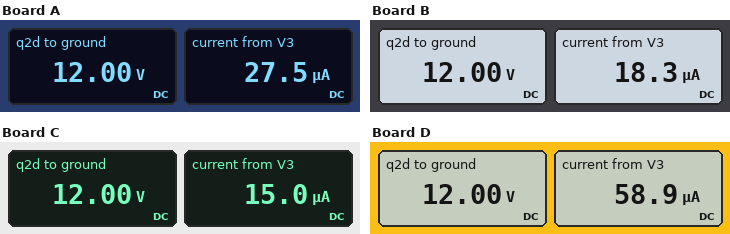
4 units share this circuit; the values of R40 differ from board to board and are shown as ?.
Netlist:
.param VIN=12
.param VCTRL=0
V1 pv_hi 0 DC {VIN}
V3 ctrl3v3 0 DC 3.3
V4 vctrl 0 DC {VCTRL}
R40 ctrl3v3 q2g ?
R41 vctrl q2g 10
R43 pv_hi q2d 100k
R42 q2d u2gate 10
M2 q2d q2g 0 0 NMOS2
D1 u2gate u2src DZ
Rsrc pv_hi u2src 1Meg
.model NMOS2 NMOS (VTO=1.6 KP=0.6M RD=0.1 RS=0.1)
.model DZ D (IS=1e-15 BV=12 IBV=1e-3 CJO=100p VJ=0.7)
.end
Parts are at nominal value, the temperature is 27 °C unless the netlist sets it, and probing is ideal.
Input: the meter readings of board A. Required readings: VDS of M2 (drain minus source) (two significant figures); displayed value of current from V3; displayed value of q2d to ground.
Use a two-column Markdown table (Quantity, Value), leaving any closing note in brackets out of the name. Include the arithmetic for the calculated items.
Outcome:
| Quantity | Value |
|---|---|
| VDS of M2 (drain minus source) | 12 V = 12 V |
| displayed value of current from V3 | 27.5 µA |
| displayed value of q2d to ground | 12.00 V |
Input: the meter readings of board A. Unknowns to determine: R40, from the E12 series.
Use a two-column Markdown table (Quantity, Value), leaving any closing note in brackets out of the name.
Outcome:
| Quantity | Value |
|---|---|
| R40, from the E12 series | 120 kΩ |
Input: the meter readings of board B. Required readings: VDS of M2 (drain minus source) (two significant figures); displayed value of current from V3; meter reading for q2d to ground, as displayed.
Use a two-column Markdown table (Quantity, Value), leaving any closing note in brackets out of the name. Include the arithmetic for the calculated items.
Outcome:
| Quantity | Value |
|---|---|
| VDS of M2 (drain minus source) | 12 V = 12 V |
| displayed value of current from V3 | 18.3 µA |
| meter reading for q2d to ground, as displayed | 12.00 V |
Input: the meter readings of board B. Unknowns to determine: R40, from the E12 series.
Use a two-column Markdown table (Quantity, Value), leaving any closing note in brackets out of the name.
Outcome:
| Quantity | Value |
|---|---|
| R40, from the E12 series | 180 kΩ |
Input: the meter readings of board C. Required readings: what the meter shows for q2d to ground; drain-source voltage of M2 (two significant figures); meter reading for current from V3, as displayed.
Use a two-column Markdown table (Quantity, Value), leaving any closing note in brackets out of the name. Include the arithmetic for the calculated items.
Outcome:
| Quantity | Value |
|---|---|
| what the meter shows for q2d to ground | 12.00 V |
| drain-source voltage of M2 | 12 V = 12 V |
| meter reading for current from V3, as displayed | 15.0 µA |
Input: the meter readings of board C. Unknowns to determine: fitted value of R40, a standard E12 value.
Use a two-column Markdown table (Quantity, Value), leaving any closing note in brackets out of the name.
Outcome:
| Quantity | Value |
|---|---|
| fitted value of R40, a standard E12 value | 220 kΩ |
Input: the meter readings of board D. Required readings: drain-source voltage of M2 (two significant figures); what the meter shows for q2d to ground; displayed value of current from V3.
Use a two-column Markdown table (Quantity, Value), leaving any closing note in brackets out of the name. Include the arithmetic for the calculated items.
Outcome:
| Quantity | Value |
|---|---|
| drain-source voltage of M2 | 12 V = 12 V |
| what the meter shows for q2d to ground | 12.00 V |
| displayed value of current from V3 | 58.9 µA |
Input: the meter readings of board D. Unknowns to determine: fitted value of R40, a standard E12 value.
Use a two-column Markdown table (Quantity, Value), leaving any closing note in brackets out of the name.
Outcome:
| Quantity | Value |
|---|---|
| fitted value of R40, a standard E12 value | 56 kΩ |
